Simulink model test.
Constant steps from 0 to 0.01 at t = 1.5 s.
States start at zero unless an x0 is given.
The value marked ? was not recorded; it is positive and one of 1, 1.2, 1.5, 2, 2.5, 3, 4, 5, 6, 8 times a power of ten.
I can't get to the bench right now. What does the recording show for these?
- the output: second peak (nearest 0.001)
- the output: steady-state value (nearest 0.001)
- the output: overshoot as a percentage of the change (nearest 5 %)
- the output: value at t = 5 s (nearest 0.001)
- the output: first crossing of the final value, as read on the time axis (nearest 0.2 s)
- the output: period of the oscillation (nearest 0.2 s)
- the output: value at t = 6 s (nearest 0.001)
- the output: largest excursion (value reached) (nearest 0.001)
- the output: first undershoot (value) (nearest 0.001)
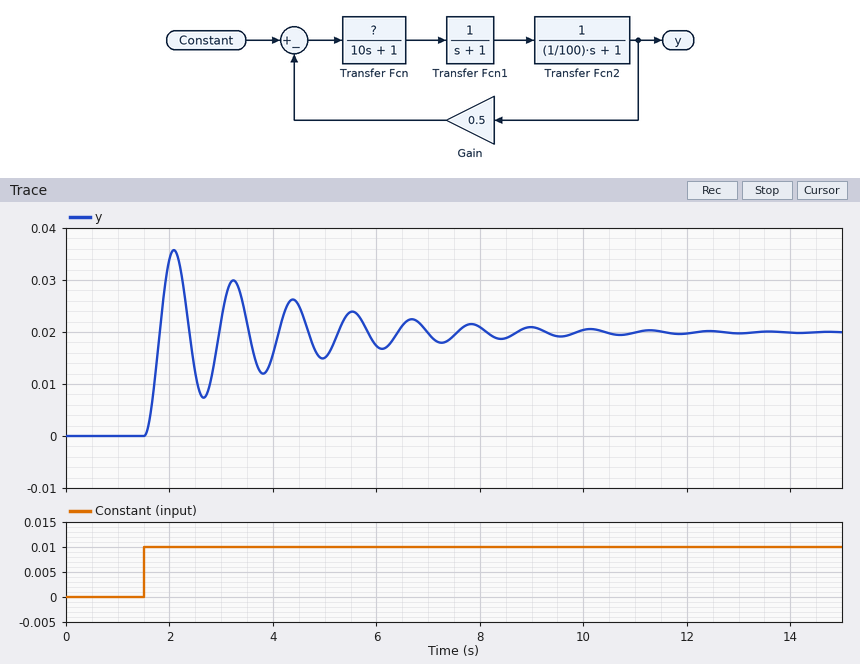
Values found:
0.030
0.020
80 %
0.015
1.8 s
1.2 s
0.017
0.036
0.007
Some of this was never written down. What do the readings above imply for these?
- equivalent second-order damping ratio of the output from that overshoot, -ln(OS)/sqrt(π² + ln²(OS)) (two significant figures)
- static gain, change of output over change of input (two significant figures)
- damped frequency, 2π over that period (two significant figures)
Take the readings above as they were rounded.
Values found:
0.071
2.0
5.2 rad/s
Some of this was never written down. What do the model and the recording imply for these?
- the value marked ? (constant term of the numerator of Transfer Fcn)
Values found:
600
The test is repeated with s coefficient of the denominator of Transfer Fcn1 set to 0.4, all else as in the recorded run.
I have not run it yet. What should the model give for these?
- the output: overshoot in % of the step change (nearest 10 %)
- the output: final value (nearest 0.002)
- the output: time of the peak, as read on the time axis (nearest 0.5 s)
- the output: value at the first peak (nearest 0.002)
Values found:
70 %
0.020
2.0 s
0.034
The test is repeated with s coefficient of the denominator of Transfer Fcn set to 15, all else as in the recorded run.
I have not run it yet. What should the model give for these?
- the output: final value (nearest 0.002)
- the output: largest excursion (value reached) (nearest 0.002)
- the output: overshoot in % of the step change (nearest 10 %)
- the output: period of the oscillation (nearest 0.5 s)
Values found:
0.020
0.034
70 %
1.5 s
